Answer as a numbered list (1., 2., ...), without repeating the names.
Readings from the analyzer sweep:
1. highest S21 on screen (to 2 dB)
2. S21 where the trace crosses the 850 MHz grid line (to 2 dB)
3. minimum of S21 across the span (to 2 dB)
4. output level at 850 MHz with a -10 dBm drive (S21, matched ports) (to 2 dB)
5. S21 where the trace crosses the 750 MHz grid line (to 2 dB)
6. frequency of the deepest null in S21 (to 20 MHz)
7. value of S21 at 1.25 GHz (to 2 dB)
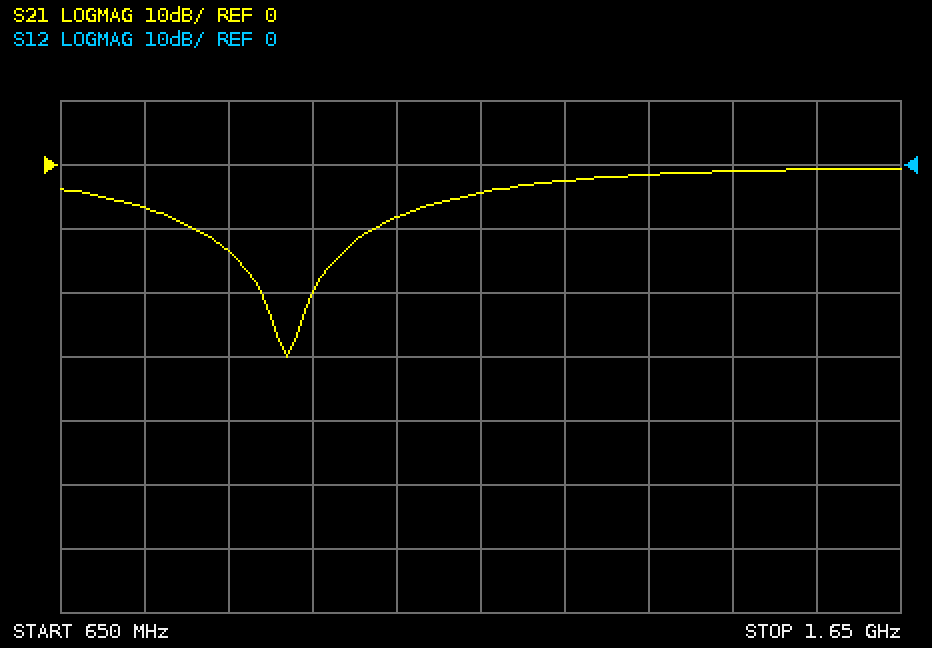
1. 0 dB
2. -14 dB
3. -30 dB
4. -24 dBm
5. -6 dB
6. 920 MHz
7. -2 dB
